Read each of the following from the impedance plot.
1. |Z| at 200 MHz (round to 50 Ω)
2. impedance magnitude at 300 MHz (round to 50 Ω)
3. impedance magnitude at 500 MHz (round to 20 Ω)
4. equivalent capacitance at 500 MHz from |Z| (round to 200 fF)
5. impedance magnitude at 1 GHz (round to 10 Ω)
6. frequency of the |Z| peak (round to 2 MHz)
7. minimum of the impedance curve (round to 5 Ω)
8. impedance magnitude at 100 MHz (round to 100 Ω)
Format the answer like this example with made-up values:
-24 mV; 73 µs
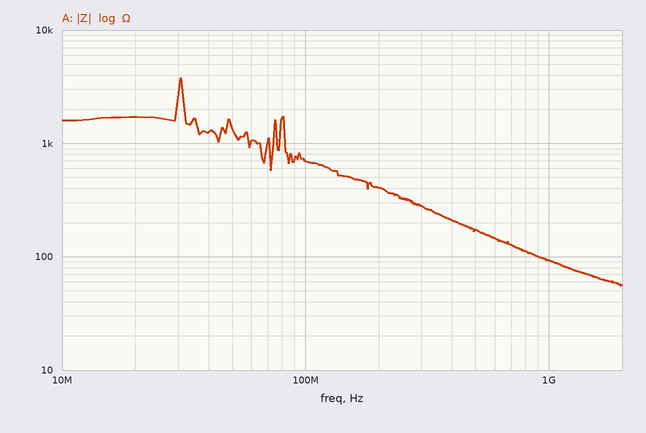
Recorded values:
400 Ω; 300 Ω; 180 Ω; 1.8 pF; 90 Ω; 30 MHz; 55 Ω; 700 Ω
